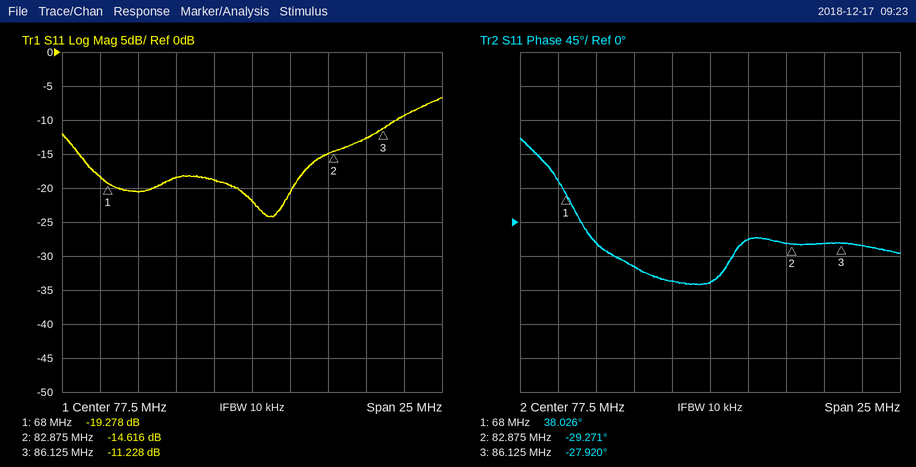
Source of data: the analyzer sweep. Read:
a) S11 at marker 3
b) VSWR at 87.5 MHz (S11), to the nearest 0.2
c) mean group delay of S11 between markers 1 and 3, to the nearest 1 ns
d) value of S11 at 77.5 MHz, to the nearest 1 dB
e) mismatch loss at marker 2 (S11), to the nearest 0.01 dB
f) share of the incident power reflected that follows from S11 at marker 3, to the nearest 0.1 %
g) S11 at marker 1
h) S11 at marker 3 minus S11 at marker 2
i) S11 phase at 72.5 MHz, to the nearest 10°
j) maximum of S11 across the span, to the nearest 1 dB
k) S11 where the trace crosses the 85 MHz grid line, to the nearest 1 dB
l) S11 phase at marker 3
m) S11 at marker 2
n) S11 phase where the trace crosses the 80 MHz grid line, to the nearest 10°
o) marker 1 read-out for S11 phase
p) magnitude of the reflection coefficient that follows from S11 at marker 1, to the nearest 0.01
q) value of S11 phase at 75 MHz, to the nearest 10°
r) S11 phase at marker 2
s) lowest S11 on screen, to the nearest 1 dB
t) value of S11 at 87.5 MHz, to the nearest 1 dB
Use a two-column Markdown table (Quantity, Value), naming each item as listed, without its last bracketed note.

| Quantity | Value |
|---|---|
| S11 at marker 3 | -11.228 dB |
| VSWR at 87.5 MHz (S11), to the nearest 0.2 | 2.0 |
| mean group delay of S11 between markers 1 and 3, to the nearest 1 ns | 10 ns |
| value of S11 at 77.5 MHz, to the nearest 1 dB | -22 dB |
| mismatch loss at marker 2 (S11), to the nearest 0.01 dB | 0.15 dB |
| share of the incident power reflected that follows from S11 at marker 3, to the nearest 0.1 % | 7.5 % |
| S11 at marker 1 | -19.278 dB |
| S11 at marker 3 minus S11 at marker 2 | 3.388 dB |
| S11 phase at 72.5 MHz, to the nearest 10° | -60° |
| maximum of S11 across the span, to the nearest 1 dB | -7 dB |
| S11 where the trace crosses the 85 MHz grid line, to the nearest 1 dB | -13 dB |
| S11 phase at marker 3 | -27.920° |
| S11 at marker 2 | -14.616 dB |
| S11 phase where the trace crosses the 80 MHz grid line, to the nearest 10° | -20° |
| marker 1 read-out for S11 phase | 38.026° |
| magnitude of the reflection coefficient that follows from S11 at marker 1, to the nearest 0.01 | 0.11 |
| value of S11 phase at 75 MHz, to the nearest 10° | -80° |
| S11 phase at marker 2 | -29.271° |
| lowest S11 on screen, to the nearest 1 dB | -24 dB |
| value of S11 at 87.5 MHz, to the nearest 1 dB | -9 dB |
